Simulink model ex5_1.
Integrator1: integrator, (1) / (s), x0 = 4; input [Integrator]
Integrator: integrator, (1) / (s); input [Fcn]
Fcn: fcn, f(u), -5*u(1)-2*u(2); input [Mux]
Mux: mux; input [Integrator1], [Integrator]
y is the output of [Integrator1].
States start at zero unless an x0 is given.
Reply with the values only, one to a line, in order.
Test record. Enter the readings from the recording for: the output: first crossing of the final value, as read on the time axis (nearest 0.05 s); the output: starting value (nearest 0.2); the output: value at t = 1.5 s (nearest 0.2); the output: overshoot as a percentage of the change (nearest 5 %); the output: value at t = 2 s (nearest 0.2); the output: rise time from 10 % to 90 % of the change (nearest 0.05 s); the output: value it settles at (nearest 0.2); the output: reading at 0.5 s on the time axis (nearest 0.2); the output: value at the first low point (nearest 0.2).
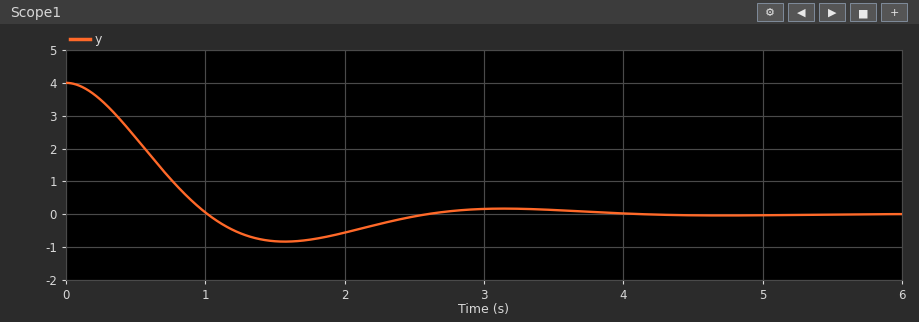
1.00 s
4.0
-0.8
20 %
-0.6
0.70 s
0.0
2.4
-0.8
